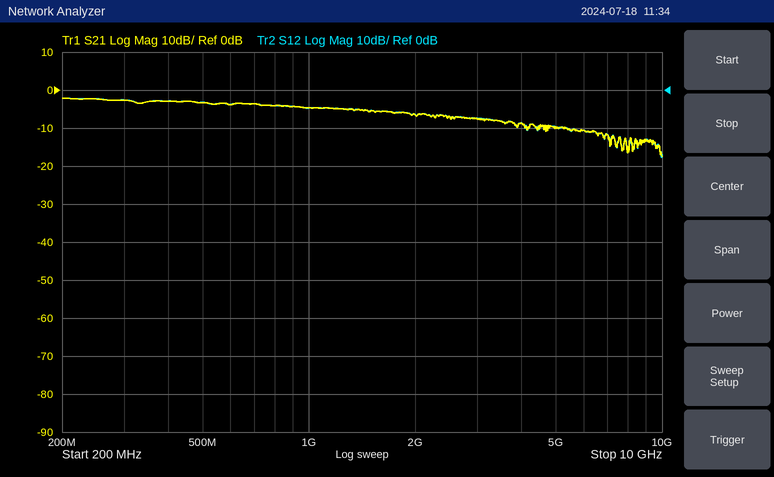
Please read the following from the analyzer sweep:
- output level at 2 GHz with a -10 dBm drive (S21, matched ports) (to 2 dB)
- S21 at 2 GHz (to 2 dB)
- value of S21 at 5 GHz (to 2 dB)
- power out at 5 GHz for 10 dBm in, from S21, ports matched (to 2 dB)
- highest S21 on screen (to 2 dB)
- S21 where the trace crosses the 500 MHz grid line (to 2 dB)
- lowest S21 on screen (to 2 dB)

-16 dBm
-6 dB
-10 dB
0 dBm
-2 dB
-4 dB
-18 dB
